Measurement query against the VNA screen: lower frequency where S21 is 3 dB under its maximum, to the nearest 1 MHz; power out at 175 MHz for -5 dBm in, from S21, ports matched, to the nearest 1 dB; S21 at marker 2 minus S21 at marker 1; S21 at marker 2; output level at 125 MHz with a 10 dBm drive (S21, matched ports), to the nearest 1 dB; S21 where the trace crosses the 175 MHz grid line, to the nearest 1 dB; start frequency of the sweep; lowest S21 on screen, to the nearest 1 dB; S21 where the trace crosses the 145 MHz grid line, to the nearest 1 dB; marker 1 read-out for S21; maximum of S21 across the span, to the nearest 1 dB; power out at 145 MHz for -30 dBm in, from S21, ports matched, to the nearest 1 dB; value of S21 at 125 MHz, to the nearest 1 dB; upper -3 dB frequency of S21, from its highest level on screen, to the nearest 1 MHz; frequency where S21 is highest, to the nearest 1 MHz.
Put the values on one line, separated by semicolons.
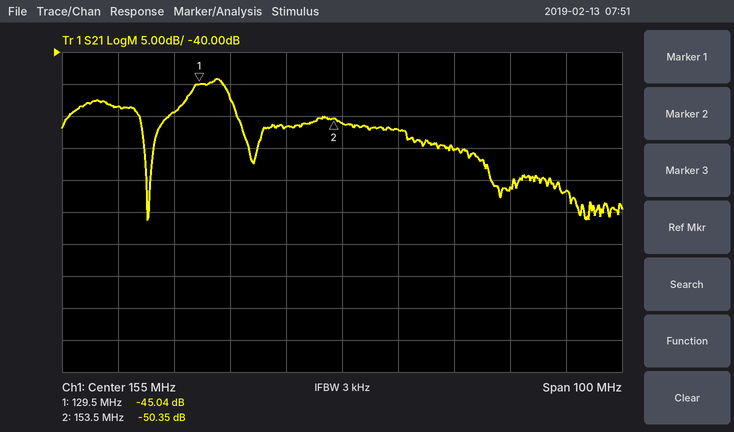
127 MHz; -60 dBm; -5.31 dB; -50.35 dB; -39 dBm; -55 dB; 105 MHz; -66 dB; -52 dB; -45.04 dB; -44 dB; -82 dBm; -49 dB; 135 MHz; 133 MHz
